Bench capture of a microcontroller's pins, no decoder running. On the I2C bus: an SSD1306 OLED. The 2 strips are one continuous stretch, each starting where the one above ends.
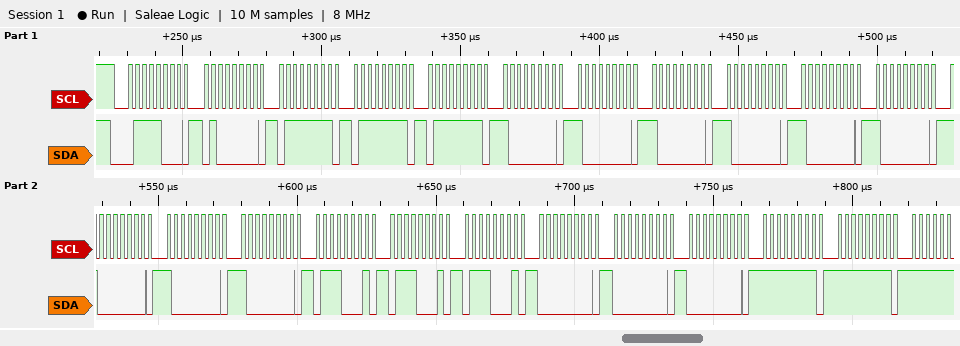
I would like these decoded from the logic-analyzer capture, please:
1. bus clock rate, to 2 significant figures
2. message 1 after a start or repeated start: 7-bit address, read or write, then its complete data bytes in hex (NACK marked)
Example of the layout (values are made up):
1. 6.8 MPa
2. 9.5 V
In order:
1. 400 kHz
2. 0x3C write: 40 7F 7F 7F 80 80 80 80 80 80 80 80 80 71 71 71 00 00 00 FF FF
